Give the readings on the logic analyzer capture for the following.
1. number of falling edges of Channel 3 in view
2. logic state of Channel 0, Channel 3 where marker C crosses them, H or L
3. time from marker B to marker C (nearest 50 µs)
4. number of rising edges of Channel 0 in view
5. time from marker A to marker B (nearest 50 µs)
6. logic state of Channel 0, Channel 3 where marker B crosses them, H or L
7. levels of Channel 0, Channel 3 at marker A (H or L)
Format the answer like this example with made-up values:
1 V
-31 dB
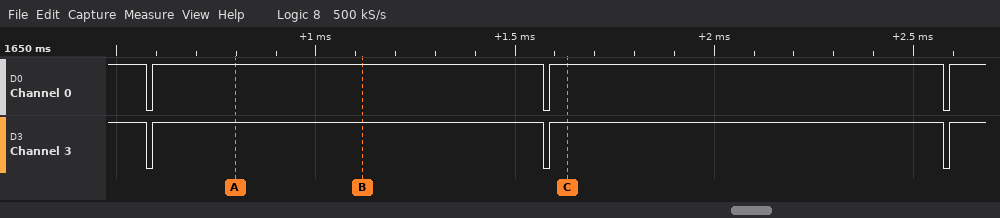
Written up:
3
Channel 0=H, Channel 3=H
500 µs
3
300 µs
Channel 0=H, Channel 3=H
Channel 0=H, Channel 3=H
